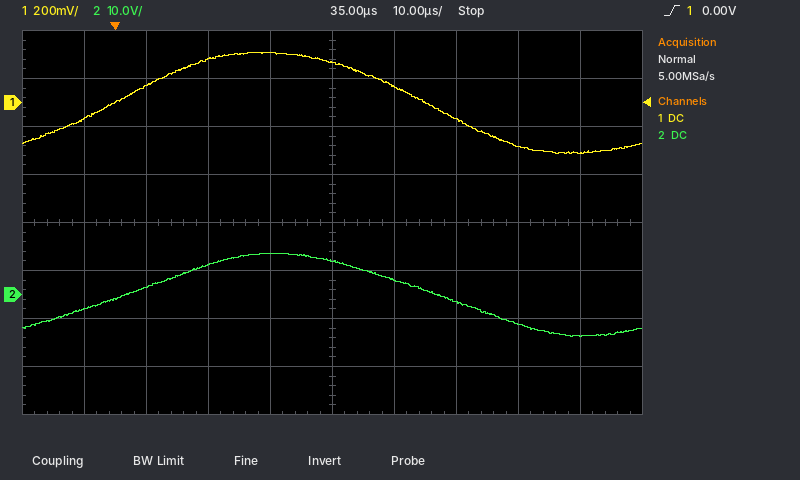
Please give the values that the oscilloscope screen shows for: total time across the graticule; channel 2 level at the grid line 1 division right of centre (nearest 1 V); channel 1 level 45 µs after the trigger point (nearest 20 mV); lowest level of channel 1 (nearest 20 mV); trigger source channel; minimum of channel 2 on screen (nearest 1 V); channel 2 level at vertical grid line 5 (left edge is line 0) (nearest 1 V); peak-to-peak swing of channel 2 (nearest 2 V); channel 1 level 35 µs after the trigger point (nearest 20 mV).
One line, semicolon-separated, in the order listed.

100 µs; 3 V; 60 mV; -220 mV; channel 1; -9 V; 7 V; 18 V; 160 mV
